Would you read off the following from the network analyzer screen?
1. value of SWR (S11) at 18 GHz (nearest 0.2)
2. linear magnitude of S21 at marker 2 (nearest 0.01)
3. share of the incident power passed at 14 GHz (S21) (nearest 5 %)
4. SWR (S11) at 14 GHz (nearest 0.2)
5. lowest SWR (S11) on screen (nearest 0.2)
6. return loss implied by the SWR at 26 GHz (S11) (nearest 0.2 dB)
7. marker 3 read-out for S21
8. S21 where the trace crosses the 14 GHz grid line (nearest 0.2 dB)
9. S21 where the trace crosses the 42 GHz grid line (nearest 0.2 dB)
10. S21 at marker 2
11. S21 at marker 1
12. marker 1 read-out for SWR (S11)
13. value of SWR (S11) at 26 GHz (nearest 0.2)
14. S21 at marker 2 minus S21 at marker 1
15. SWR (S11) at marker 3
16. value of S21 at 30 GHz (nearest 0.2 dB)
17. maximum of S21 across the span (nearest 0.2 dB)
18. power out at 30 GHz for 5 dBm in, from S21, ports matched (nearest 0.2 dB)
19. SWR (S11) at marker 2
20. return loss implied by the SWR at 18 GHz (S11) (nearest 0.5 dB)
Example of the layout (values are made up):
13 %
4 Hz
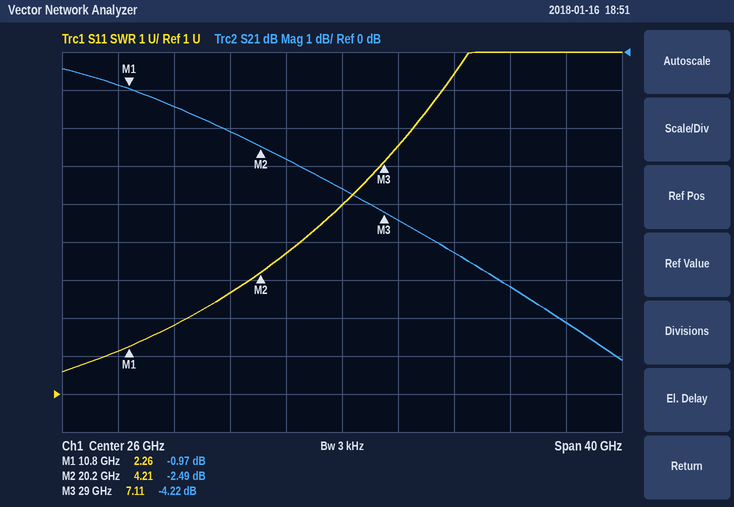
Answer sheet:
3.6
0.75
70 %
2.8
1.6
3.0 dB
-4.22 dB
-1.4 dB
-7.2 dB
-2.49 dB
-0.97 dB
2.26
6.0
-1.52 dB
7.11
-4.4 dB
-0.4 dB
0.6 dBm
4.21
5.0 dB
